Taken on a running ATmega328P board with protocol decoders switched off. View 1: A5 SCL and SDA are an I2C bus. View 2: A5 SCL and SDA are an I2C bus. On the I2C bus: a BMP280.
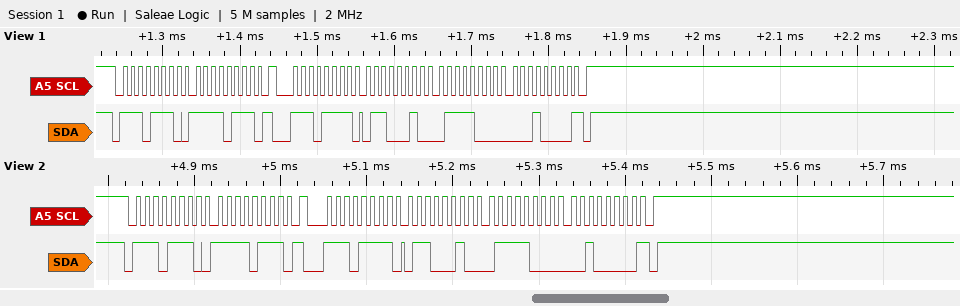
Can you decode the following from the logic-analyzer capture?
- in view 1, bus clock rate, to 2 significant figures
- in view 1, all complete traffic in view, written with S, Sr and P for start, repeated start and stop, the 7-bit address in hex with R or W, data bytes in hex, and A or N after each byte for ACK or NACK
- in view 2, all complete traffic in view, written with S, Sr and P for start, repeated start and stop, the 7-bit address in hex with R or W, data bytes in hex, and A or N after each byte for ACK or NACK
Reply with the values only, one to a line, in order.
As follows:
100 kHz
S 77W A F7 A Sr 77R A 62 A 78 A 10 N P
S 77W A F7 A Sr 77R A 62 A 78 A 20 N P
